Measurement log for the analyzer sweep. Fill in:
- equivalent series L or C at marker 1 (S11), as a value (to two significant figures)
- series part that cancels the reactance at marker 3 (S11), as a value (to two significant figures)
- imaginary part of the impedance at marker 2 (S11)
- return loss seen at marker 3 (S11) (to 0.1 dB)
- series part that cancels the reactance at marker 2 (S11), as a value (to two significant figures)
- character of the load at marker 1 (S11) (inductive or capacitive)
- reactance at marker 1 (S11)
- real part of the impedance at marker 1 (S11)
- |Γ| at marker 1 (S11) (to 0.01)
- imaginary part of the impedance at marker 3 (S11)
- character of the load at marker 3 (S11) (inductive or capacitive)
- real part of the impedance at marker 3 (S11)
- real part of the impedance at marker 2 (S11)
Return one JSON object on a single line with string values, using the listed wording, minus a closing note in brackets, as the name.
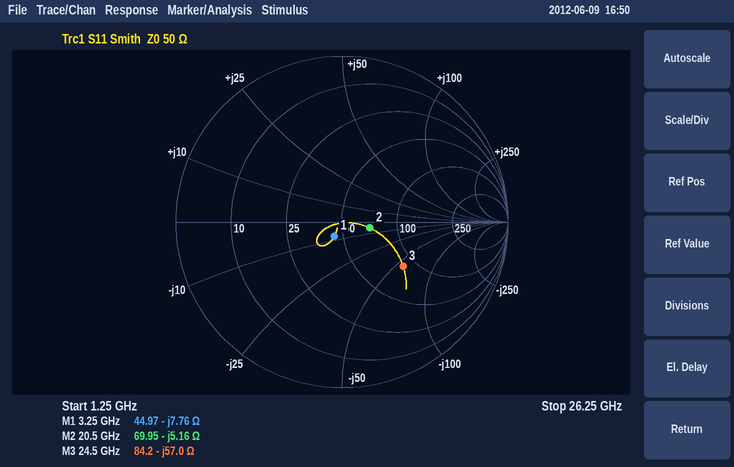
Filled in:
{"equivalent series L or C at marker 1 (S11), as a value": "6.3 pF", "series part that cancels the reactance at marker 3 (S11), as a value": "370 pH", "imaginary part of the impedance at marker 2": "-5.16 Ω", "return loss seen at marker 3 (S11)": "6.8 dB", "series part that cancels the reactance at marker 2 (S11), as a value": "40 pH", "character of the load at marker 1 (S11)": "capacitive", "reactance at marker 1": "-7.76 Ω", "real part of the impedance at marker 1": "44.97 Ω", "|Γ| at marker 1 (S11)": "0.10", "imaginary part of the impedance at marker 3": "-57.0 Ω", "character of the load at marker 3 (S11)": "capacitive", "real part of the impedance at marker 3": "84.2 Ω", "real part of the impedance at marker 2": "69.95 Ω"}
